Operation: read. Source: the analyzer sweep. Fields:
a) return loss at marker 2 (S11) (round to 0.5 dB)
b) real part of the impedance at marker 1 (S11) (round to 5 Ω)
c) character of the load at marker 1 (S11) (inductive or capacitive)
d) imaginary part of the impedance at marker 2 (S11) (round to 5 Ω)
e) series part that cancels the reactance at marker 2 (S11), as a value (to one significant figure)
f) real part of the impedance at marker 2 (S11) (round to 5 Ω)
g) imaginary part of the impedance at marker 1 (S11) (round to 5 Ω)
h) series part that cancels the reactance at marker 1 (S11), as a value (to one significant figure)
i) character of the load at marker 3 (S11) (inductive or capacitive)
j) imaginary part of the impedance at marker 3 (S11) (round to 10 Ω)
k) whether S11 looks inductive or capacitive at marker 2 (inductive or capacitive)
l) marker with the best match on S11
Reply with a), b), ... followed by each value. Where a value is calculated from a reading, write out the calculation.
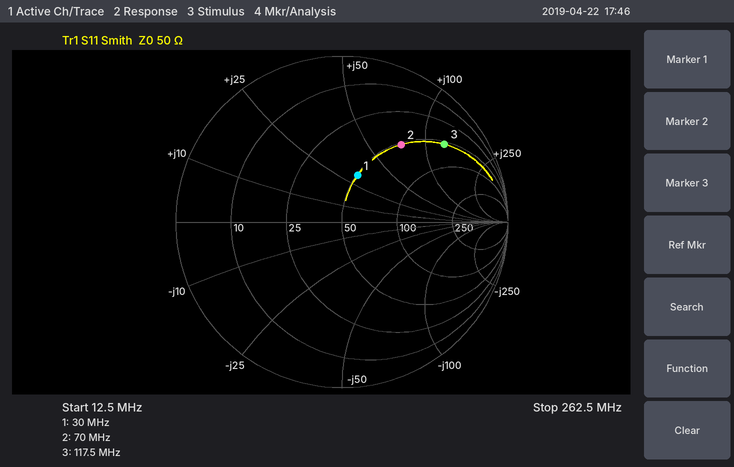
a) 4.5 dB
b) 50 Ω
c) inductive
d) +75 Ω
e) C = 1/(2π × 70 MHz × 75 Ω) ≈ 30 pF
f) 50 Ω
g) +30 Ω
h) C = 1/(2π × 30 MHz × 30 Ω) ≈ 177 pF, so 200 pF to one significant figure
i) inductive
j) +130 Ω
k) inductive
l) marker 1
